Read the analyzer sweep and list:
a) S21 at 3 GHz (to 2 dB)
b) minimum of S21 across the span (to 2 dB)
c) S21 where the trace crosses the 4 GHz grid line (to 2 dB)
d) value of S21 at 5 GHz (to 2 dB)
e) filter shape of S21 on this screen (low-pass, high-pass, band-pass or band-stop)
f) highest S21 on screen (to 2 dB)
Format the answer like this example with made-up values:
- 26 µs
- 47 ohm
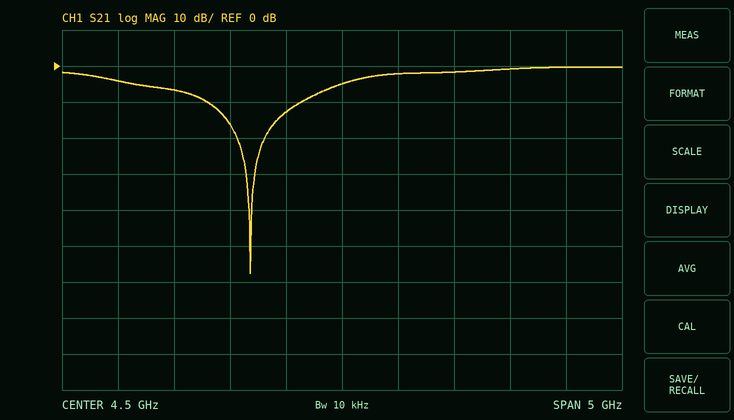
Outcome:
- -6 dB
- -58 dB
- -12 dB
- -2 dB
- band-stop
- 0 dB
